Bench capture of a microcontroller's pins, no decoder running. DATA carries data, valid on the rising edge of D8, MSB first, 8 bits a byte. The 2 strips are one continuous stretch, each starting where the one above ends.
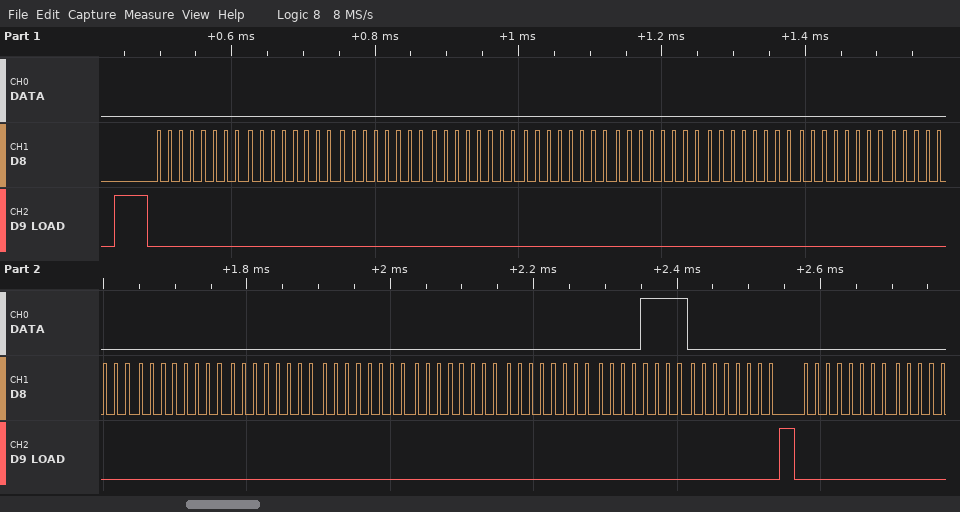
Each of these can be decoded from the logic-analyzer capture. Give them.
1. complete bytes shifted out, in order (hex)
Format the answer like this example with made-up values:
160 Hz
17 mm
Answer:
0x00 0x00 0x00 0x00 0x00 0x00 0x00 0x00 0x00 0x00 0x00 0x00 0x00 0x00 0x0F 0x00 0x00
